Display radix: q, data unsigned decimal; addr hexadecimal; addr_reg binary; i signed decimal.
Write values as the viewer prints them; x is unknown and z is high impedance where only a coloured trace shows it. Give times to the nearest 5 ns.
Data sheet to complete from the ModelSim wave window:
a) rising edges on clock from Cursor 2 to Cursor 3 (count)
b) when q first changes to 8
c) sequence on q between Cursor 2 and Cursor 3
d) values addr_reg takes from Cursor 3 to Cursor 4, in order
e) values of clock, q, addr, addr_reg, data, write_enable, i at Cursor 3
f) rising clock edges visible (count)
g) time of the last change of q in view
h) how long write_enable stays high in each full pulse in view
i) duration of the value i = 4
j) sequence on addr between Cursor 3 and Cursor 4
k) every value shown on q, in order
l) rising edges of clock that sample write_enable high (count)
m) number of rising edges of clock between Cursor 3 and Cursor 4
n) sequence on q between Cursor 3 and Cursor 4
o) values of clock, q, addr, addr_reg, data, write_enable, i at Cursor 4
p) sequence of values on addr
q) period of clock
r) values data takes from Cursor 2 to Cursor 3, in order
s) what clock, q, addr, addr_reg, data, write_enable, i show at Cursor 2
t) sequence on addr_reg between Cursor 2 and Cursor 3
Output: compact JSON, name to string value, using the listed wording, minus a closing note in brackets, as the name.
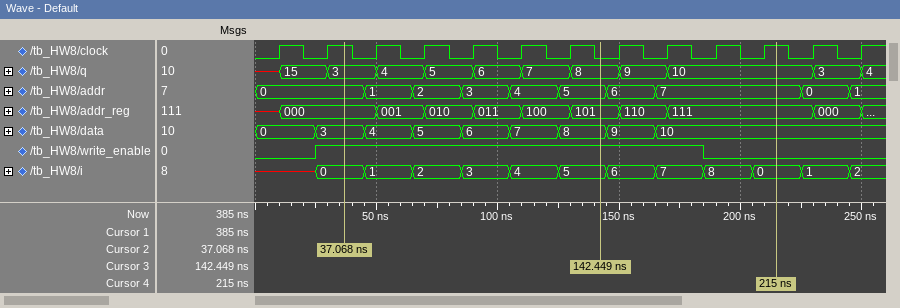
{"rising edges on clock from Cursor 2 to Cursor 3": "5", "when q first changes to 8": "130 ns", "sequence on q between Cursor 2 and Cursor 3": "3, 4, 5, 6, 7, 8", "values addr_reg takes from Cursor 3 to Cursor 4, in order": "101, 110, 111", "values of clock, q, addr, addr_reg, data, write_enable, i at Cursor 3": "clock=0, q=8, addr=5, addr_reg=101, data=8, write_enable=1, i=5", "rising clock edges visible": "13", "time of the last change of q in view": "250 ns", "how long write_enable stays high in each full pulse in view": "160 ns", "duration of the value i = 4": "20 ns", "sequence on addr between Cursor 3 and Cursor 4": "5, 6, 7", "every value shown on q, in order": "x, 15, 3, 4, 5, 6, 7, 8, 9, 10, 3, 4", "rising edges of clock that sample write_enable high": "8", "number of rising edges of clock between Cursor 3 and Cursor 4": "4", "sequence on q between Cursor 3 and Cursor 4": "8, 9, 10", "values of clock, q, addr, addr_reg, data, write_enable, i at Cursor 4": "clock=1, q=10, addr=7, addr_reg=111, data=10, write_enable=0, i=0", "sequence of values on addr": "0, 1, 2, 3, 4, 5, 6, 7, 0, 1", "period of clock": "20 ns", "values data takes from Cursor 2 to Cursor 3, in order": "3, 4, 5, 6, 7, 8", "what clock, q, addr, addr_reg, data, write_enable, i show at Cursor 2": "clock=1, q=3, addr=0, addr_reg=000, data=3, write_enable=1, i=0", "sequence on addr_reg between Cursor 2 and Cursor 3": "000, 001, 010, 011, 100, 101"}
